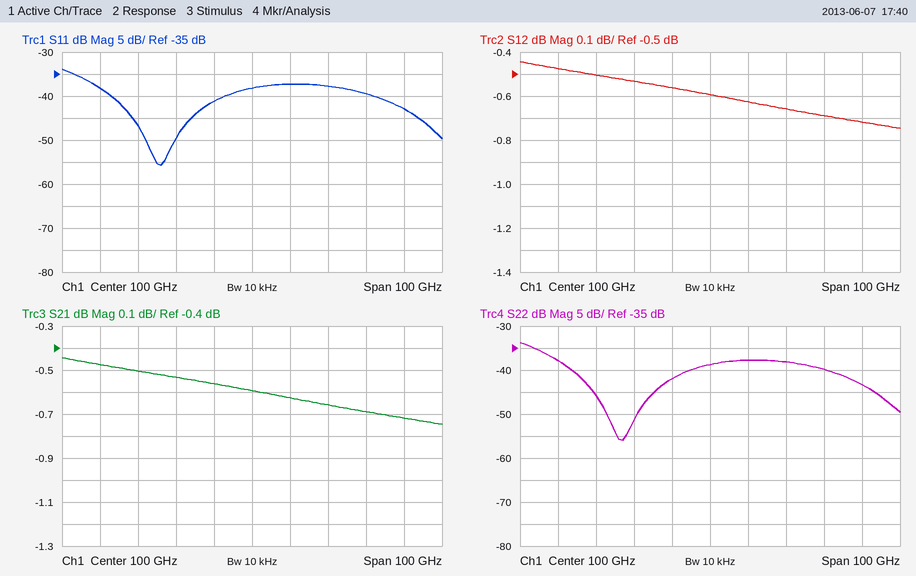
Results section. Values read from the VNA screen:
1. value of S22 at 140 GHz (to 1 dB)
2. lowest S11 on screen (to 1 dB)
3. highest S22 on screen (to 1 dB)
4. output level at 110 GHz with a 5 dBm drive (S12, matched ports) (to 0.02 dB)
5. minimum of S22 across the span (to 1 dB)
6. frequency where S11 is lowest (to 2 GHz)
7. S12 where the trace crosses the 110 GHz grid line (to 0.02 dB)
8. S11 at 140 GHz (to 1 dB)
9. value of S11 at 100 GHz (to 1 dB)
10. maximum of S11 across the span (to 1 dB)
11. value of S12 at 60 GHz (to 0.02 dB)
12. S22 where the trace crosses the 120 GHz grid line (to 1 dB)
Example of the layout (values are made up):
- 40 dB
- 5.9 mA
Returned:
- -43 dB
- -56 dB
- -34 dB
- 4.38 dBm
- -56 dB
- 76 GHz
- -0.62 dB
- -43 dB
- -38 dB
- -34 dB
- -0.48 dB
- -38 dB
